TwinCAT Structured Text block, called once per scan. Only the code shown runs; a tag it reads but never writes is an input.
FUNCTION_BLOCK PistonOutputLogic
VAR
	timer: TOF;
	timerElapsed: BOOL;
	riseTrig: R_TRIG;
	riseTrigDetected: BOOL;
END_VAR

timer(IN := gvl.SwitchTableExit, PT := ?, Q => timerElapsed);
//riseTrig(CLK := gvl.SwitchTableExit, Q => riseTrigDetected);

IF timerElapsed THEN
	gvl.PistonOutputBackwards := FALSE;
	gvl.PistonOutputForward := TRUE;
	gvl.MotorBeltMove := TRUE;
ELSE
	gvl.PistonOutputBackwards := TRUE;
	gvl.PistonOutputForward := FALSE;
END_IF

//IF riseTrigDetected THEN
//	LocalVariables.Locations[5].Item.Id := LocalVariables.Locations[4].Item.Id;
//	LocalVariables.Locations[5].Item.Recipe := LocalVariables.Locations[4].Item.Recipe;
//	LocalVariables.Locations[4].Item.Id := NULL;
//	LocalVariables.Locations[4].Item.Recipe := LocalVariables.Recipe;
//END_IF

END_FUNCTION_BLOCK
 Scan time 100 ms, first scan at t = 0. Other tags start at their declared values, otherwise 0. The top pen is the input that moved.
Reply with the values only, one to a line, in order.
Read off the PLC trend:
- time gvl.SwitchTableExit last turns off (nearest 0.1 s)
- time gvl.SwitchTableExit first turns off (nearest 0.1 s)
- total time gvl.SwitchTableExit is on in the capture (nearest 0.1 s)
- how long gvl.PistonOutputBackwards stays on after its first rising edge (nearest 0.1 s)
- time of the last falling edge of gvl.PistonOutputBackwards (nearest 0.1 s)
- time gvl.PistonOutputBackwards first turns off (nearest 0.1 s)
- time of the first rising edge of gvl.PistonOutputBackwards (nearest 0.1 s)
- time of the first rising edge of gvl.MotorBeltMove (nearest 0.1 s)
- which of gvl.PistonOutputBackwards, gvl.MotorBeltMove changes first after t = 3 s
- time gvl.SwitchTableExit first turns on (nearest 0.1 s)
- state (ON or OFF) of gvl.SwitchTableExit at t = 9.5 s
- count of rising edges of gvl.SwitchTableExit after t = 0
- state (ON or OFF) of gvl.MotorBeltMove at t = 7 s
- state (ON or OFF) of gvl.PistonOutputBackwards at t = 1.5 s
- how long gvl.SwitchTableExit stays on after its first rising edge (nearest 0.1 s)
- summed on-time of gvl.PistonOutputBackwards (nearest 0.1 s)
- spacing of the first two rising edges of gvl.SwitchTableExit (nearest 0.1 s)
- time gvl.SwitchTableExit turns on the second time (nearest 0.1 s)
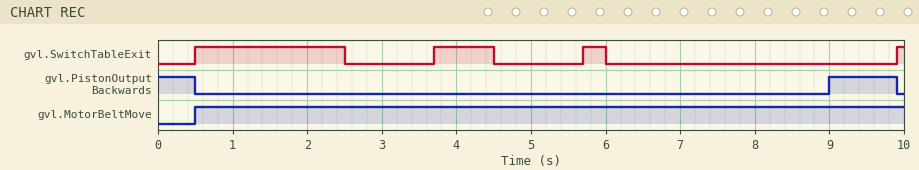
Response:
6.0 s
2.5 s
3.2 s
0.9 s
9.9 s
0.5 s
9.0 s
0.5 s
gvl.PistonOutputBackwards
0.5 s
OFF
4
ON
OFF
2.0 s
1.4 s
3.2 s
3.7 s
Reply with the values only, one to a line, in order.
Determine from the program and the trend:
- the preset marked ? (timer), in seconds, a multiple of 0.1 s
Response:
3.0 s
